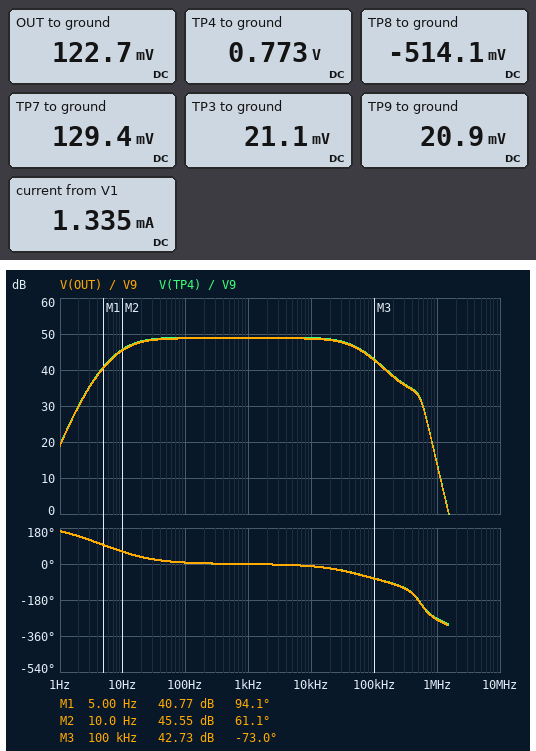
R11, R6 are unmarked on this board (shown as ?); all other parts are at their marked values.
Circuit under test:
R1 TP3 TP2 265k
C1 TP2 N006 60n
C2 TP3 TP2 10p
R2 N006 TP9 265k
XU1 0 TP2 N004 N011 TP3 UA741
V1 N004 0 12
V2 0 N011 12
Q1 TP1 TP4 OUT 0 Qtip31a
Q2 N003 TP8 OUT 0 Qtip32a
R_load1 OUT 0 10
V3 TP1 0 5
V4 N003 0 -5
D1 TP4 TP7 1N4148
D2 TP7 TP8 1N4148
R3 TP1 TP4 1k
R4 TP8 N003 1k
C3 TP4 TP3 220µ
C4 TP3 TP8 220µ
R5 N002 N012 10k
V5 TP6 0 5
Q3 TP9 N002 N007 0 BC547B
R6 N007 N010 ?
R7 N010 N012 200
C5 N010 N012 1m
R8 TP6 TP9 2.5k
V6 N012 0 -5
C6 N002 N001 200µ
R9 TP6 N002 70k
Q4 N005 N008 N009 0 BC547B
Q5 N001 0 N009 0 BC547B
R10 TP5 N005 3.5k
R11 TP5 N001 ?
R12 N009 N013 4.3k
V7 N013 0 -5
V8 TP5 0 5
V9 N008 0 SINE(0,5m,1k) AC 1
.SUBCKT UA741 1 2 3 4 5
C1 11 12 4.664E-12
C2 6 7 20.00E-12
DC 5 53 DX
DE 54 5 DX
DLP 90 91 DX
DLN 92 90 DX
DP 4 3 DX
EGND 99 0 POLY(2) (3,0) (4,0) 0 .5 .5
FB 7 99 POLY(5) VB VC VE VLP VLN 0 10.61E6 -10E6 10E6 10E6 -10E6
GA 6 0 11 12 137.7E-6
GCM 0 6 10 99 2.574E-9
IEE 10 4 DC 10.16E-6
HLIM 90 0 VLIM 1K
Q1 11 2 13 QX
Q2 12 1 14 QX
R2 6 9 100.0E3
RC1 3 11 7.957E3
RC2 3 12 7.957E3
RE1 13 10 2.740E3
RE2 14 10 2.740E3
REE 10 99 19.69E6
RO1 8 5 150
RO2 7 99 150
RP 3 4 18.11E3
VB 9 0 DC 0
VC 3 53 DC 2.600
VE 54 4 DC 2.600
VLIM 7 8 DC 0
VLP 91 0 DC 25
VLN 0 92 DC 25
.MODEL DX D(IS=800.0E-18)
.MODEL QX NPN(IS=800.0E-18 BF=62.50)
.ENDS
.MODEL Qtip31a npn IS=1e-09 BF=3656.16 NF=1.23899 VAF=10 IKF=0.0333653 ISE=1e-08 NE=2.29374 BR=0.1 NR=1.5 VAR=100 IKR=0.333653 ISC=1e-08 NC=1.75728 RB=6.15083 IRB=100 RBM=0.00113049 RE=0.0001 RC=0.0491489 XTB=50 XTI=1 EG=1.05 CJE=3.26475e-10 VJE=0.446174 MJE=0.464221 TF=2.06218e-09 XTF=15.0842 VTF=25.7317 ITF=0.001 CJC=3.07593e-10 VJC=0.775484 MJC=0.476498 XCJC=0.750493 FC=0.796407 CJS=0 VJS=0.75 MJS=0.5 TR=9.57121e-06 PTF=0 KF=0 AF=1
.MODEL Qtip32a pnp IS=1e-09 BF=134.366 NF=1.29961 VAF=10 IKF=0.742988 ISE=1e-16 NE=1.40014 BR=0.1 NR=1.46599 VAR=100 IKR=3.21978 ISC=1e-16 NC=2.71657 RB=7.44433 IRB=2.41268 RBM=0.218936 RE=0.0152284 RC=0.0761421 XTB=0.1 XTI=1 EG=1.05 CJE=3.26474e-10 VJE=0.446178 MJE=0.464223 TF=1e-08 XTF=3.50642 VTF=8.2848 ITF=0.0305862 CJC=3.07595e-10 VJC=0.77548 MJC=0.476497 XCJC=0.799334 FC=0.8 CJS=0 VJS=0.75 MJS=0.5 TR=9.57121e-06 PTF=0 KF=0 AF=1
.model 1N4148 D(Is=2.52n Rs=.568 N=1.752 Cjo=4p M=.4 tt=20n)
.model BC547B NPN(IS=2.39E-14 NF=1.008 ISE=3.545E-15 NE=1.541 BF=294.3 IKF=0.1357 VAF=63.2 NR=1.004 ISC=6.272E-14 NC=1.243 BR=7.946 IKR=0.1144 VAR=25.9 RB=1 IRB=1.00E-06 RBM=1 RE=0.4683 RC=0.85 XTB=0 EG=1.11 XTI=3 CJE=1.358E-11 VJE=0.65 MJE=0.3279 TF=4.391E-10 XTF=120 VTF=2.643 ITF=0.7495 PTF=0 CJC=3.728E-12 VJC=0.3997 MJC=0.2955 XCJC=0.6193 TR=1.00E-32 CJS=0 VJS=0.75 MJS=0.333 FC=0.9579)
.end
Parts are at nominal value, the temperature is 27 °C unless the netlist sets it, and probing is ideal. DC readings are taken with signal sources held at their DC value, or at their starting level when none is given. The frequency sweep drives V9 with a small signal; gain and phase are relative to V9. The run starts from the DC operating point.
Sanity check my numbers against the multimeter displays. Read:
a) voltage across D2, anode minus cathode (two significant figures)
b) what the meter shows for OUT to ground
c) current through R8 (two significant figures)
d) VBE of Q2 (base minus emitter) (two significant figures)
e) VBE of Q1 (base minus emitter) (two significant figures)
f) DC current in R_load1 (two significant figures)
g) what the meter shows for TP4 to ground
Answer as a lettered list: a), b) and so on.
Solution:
a) 640 mV
b) 122.7 mV
c) 2.0 mA
d) -640 mV
e) 650 mV
f) 12 mA
g) 0.773 V
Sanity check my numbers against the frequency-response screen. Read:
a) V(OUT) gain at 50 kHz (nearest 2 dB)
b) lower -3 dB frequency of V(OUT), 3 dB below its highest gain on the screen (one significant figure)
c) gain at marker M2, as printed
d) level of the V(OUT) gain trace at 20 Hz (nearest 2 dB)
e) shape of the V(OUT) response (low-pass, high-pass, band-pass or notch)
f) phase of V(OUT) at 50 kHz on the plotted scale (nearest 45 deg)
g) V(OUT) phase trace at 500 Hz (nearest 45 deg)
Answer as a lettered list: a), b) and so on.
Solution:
a) 46 dB
b) 10 Hz
c) 45.55 dB
d) 48 dB
e) band-pass
f) -45 deg
g) 0 deg
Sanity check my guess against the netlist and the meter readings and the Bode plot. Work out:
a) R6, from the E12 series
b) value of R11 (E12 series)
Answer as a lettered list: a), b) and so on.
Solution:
a) 68 Ω
b) 1.2 kΩ
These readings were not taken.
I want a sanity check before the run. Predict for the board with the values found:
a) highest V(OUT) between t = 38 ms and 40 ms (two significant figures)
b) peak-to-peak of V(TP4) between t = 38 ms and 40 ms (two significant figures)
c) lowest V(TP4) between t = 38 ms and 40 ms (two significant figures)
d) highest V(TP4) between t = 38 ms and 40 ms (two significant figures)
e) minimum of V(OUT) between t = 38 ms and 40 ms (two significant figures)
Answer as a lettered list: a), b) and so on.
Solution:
a) 1.5 V
b) 2.8 V
c) -610 mV
d) 2.2 V
e) -1.2 V
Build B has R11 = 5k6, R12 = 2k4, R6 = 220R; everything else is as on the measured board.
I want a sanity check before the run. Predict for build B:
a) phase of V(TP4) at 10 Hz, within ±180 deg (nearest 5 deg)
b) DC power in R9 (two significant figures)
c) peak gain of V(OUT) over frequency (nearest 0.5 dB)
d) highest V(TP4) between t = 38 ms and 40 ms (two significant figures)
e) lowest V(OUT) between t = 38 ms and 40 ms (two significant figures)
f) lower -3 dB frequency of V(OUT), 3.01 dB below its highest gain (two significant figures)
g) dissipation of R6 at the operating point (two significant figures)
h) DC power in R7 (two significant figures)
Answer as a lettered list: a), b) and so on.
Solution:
a) 55 deg
b) 1.1 mW
c) 54.5 dB
d) 3.4 V
e) -2.4 V
f) 10 Hz
g) 400 µW
h) 360 µW
